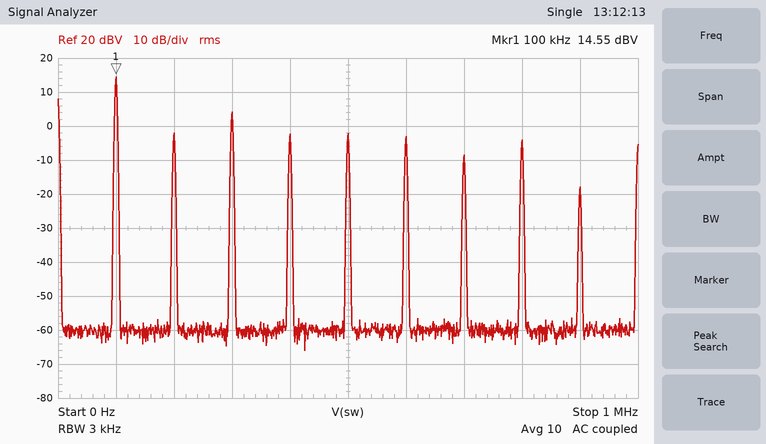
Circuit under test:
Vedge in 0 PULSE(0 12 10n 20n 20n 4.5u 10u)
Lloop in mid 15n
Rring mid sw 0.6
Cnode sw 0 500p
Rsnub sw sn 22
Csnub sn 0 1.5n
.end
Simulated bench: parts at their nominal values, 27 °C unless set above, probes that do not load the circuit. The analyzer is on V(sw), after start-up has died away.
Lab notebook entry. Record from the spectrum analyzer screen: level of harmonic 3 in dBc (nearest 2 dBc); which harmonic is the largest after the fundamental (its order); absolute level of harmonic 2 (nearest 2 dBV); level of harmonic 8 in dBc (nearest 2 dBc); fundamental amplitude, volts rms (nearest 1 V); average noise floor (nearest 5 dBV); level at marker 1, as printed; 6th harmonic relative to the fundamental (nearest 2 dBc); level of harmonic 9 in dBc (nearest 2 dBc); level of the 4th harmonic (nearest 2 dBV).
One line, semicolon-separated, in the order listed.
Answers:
-10 dBc; 3; -2 dBV; -18 dBc; 5 V; -60 dBV; 14.55 dBV; -18 dBc; -32 dBc; -2 dBV
